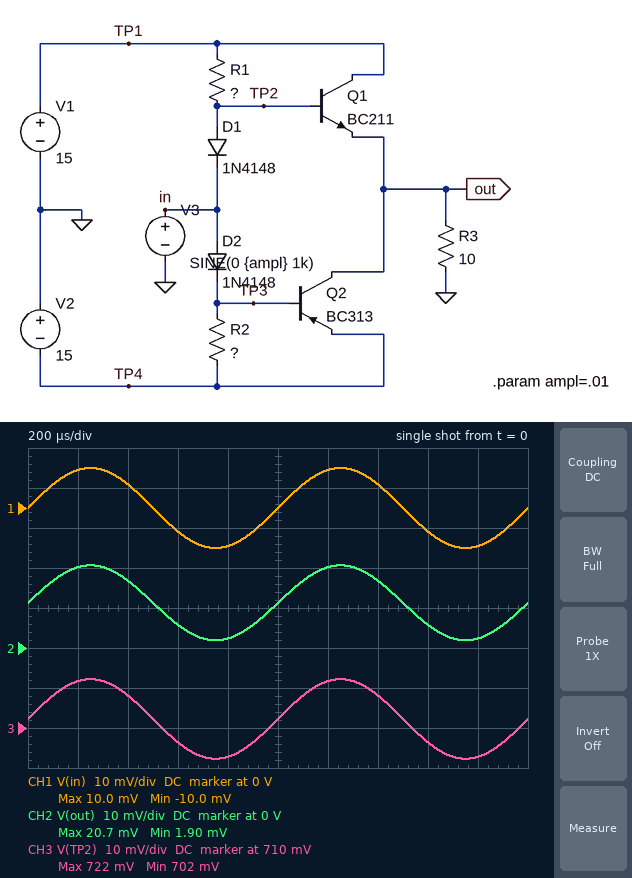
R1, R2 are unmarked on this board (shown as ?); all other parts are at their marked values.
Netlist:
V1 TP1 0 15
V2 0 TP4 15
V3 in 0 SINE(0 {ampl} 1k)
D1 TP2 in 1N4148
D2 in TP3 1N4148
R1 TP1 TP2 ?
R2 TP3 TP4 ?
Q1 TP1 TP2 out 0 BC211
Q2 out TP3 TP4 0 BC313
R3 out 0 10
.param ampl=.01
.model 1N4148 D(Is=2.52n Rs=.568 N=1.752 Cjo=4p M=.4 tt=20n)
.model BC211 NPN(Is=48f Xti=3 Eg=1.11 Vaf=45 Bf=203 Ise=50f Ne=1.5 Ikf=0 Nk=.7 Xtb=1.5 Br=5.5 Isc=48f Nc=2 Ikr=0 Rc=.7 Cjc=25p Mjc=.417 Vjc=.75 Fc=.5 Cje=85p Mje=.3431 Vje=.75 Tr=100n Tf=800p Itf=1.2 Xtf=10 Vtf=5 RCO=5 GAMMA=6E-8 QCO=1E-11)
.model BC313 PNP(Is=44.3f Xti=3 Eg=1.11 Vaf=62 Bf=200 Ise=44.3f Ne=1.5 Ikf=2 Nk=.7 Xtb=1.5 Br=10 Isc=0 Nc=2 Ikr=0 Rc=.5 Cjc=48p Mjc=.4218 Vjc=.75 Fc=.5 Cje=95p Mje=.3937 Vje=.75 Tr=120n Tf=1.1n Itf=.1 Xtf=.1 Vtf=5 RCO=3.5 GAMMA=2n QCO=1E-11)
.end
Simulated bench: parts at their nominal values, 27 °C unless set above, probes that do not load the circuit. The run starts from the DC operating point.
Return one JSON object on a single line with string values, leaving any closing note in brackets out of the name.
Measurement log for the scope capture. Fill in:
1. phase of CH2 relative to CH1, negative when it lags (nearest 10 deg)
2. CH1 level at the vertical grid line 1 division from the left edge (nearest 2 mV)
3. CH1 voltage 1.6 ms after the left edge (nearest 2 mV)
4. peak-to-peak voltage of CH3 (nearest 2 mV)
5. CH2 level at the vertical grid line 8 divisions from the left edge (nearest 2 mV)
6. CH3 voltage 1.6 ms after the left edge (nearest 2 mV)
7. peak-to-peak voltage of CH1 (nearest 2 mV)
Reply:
{"phase of CH2 relative to CH1, negative when it lags": "0 deg", "CH1 level at the vertical grid line 1 division from the left edge": "10 mV", "CH1 voltage 1.6 ms after the left edge": "-6 mV", "peak-to-peak voltage of CH3": "20 mV", "CH2 level at the vertical grid line 8 divisions from the left edge": "6 mV", "CH3 voltage 1.6 ms after the left edge": "706 mV", "peak-to-peak voltage of CH1": "20 mV"}
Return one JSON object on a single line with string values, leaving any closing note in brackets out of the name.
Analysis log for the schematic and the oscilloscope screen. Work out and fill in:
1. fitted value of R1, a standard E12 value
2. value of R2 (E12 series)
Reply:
{"fitted value of R1, a standard E12 value": "1 kΩ", "value of R2": "150 Ω"}
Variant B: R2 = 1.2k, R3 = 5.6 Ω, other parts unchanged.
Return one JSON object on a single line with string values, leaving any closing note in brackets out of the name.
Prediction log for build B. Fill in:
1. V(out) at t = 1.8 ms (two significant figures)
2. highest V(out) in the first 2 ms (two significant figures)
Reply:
{"V(out) at t = 1.8 ms": "23 mV", "highest V(out) in the first 2 ms": "39 mV"}
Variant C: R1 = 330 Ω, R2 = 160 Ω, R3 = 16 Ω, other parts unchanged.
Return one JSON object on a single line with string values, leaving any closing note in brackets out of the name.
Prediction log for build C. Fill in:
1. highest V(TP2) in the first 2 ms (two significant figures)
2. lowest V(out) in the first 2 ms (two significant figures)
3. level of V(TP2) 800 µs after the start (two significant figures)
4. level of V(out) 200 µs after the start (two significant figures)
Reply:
{"highest V(TP2) in the first 2 ms": "790 mV", "lowest V(out) in the first 2 ms": "60 mV", "level of V(TP2) 800 µs after the start": "770 mV", "level of V(out) 200 µs after the start": "79 mV"}
